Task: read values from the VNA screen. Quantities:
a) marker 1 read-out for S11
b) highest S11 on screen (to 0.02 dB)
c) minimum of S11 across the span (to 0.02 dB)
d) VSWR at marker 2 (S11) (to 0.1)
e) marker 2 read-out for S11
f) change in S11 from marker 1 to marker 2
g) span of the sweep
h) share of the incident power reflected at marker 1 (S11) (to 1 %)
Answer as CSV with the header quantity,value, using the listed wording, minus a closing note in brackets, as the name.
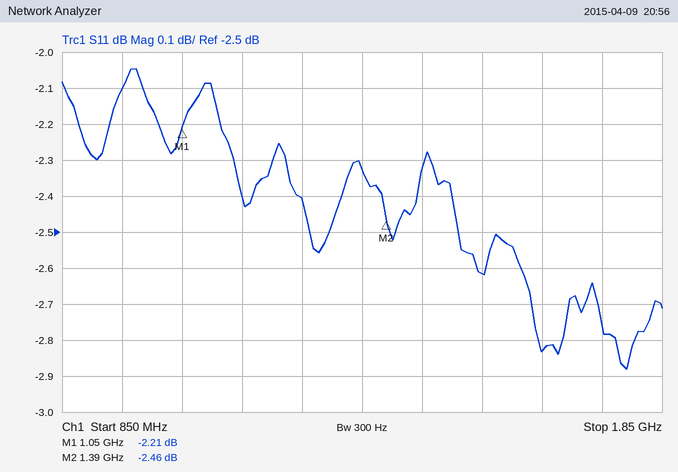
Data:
quantity,value
marker 1 read-out for S11,-2.21 dB
highest S11 on screen,-2.04 dB
minimum of S11 across the span,-2.88 dB
VSWR at marker 2 (S11),7.1
marker 2 read-out for S11,-2.46 dB
change in S11 from marker 1 to marker 2,-0.25 dB
span of the sweep,1 GHz
share of the incident power reflected at marker 1 (S11),60 %
